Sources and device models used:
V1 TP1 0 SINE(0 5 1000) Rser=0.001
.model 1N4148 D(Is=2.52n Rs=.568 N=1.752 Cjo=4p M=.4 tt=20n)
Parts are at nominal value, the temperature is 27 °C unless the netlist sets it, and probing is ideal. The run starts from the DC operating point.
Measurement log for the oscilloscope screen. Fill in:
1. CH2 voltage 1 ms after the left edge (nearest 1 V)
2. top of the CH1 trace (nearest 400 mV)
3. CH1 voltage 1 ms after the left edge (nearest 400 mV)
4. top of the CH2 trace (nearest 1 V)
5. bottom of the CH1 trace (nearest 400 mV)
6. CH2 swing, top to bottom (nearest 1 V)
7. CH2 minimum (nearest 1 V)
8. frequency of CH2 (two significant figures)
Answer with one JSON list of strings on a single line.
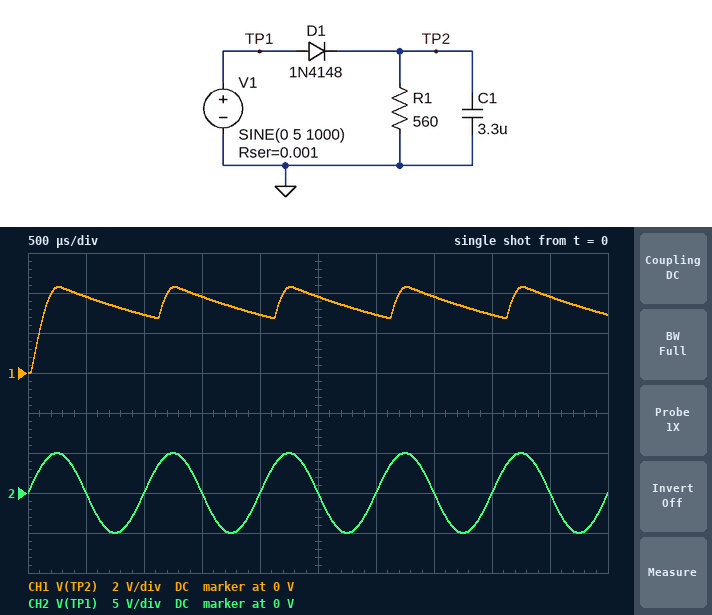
["0 V", "4.4 V", "2.8 V", "5 V", "0 V", "10 V", "-5 V", "1.0 kHz"]
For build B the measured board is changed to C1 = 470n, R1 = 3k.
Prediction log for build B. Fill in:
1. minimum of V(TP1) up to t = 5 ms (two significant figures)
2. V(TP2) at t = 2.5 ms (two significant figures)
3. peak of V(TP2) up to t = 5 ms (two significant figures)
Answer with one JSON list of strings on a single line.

["-5.0 V", "3.7 V", "4.4 V"]
